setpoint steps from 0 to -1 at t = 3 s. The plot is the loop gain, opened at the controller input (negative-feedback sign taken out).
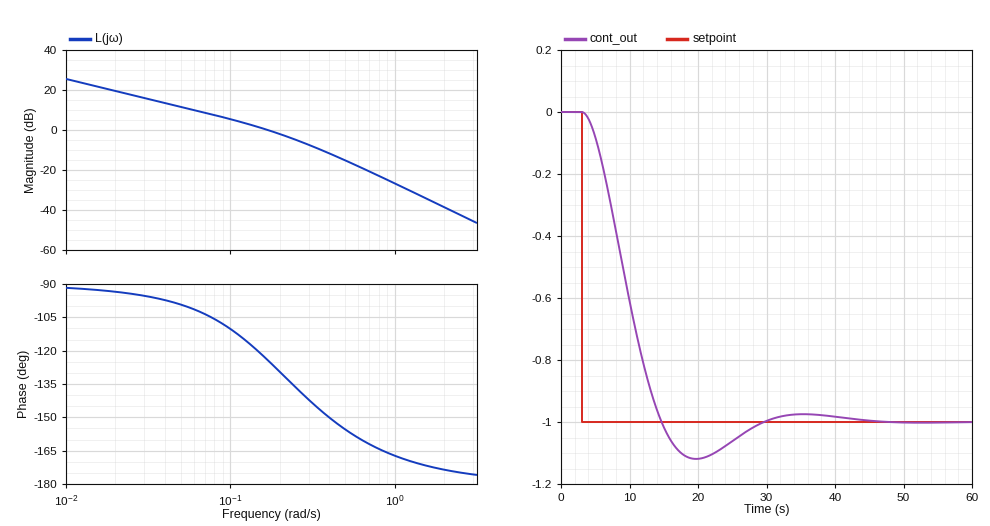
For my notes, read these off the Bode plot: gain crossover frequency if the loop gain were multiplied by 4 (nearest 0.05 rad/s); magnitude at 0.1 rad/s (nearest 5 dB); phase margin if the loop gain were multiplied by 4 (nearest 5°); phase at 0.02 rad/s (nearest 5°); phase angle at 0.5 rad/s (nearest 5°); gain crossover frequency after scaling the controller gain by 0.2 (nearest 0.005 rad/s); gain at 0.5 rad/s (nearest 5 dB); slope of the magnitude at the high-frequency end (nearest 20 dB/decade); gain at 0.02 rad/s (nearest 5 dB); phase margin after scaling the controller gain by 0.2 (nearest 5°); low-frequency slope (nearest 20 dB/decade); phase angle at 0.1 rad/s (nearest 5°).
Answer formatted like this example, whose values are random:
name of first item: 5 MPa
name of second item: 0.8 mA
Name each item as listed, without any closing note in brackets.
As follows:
gain crossover frequency if the loop gain were multiplied by 4: 0.40 rad/s
magnitude at 0.1 rad/s: 5 dB
phase margin if the loop gain were multiplied by 4: 30°
phase at 0.02 rad/s: -95°
phase angle at 0.5 rad/s: -155°
gain crossover frequency after scaling the controller gain by 0.2: 0.040 rad/s
gain at 0.5 rad/s: -15 dB
slope of the magnitude at the high-frequency end: -40 dB/decade
gain at 0.02 rad/s: 20 dB
phase margin after scaling the controller gain by 0.2: 85°
low-frequency slope: -20 dB/decade
phase angle at 0.1 rad/s: -110°
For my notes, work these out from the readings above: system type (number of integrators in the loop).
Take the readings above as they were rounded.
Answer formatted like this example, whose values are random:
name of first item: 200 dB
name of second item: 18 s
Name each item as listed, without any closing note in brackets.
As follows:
system type: 1
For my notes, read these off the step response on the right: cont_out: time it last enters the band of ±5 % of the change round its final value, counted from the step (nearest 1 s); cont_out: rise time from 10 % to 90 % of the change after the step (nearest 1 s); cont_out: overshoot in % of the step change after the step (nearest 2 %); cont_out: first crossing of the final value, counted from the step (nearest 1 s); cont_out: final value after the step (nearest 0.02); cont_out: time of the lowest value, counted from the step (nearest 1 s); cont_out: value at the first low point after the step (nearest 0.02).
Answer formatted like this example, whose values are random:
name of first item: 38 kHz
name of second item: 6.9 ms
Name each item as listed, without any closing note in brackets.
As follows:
cont_out: time it last enters the band of ±5 % of the change round its final value, counted from the step: 23 s
cont_out: rise time from 10 % to 90 % of the change after the step: 8 s
cont_out: overshoot in % of the step change after the step: 12 %
cont_out: first crossing of the final value, counted from the step: 12 s
cont_out: final value after the step: -1.00
cont_out: time of the lowest value, counted from the step: 17 s
cont_out: value at the first low point after the step: -1.12
